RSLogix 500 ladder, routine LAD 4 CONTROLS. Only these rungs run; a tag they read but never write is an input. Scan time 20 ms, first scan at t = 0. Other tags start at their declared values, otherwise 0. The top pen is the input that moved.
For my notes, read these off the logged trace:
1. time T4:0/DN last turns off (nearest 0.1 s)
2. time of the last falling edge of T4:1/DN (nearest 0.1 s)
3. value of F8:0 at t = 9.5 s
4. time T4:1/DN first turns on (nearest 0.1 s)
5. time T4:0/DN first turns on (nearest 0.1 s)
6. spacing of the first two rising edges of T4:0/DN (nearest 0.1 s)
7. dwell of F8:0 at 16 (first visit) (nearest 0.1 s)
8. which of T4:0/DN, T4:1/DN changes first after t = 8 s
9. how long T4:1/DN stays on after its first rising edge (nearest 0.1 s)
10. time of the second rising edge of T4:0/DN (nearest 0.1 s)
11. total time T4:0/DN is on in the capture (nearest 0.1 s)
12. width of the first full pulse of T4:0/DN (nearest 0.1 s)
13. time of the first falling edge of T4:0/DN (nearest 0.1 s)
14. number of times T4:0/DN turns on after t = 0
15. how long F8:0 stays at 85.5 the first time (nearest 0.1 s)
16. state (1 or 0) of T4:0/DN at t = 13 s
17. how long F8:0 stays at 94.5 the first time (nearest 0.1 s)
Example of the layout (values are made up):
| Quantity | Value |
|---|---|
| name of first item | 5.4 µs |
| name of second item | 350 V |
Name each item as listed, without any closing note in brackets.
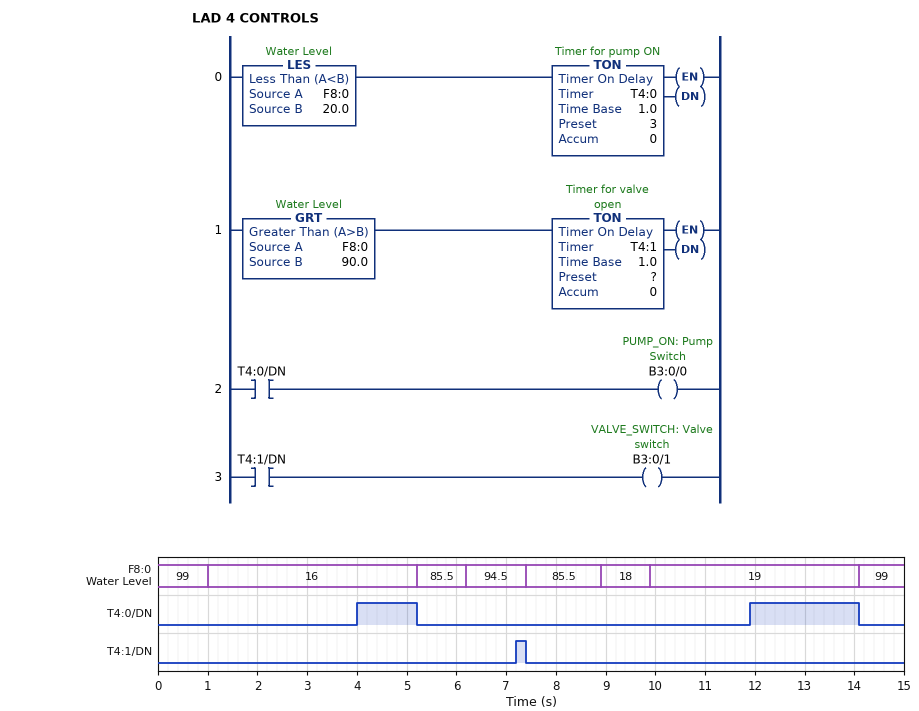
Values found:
| Quantity | Value |
|---|---|
| time T4:0/DN last turns off | 14.1 s |
| time of the last falling edge of T4:1/DN | 7.4 s |
| value of F8:0 at t = 9.5 s | 18 |
| time T4:1/DN first turns on | 7.2 s |
| time T4:0/DN first turns on | 4.0 s |
| spacing of the first two rising edges of T4:0/DN | 7.9 s |
| dwell of F8:0 at 16 (first visit) | 4.2 s |
| which of T4:0/DN, T4:1/DN changes first after t = 8 s | T4:0/DN |
| how long T4:1/DN stays on after its first rising edge | 0.2 s |
| time of the second rising edge of T4:0/DN | 11.9 s |
| total time T4:0/DN is on in the capture | 3.4 s |
| width of the first full pulse of T4:0/DN | 1.2 s |
| time of the first falling edge of T4:0/DN | 5.2 s |
| number of times T4:0/DN turns on after t = 0 | 2 |
| how long F8:0 stays at 85.5 the first time | 1.0 s |
| state (1 or 0) of T4:0/DN at t = 13 s | 1 |
| how long F8:0 stays at 94.5 the first time | 1.2 s |
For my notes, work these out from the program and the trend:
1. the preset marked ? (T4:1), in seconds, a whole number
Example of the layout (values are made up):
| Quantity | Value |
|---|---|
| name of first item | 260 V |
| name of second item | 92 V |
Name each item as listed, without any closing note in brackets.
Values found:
| Quantity | Value |
|---|---|
| the preset marked ? (T4:1), in seconds, a whole number | 1 s |
